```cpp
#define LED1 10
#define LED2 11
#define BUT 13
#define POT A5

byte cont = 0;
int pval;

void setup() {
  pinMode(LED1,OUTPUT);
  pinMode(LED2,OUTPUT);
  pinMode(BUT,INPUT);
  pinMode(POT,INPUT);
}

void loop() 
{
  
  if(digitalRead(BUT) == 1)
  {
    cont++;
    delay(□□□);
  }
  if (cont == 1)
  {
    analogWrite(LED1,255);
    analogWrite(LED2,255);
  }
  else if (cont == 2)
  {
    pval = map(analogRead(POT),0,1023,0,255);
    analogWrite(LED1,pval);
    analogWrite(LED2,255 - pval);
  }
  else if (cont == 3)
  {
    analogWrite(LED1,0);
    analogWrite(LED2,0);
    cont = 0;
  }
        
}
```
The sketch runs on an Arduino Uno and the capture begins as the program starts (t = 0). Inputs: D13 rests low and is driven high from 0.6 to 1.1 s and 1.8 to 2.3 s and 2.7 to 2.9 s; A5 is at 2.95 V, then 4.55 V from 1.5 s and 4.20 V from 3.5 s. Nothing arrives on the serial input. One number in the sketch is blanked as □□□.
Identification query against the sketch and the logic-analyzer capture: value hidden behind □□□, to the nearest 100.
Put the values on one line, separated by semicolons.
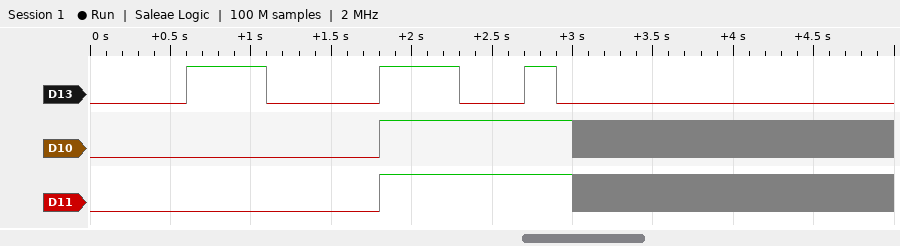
1200
